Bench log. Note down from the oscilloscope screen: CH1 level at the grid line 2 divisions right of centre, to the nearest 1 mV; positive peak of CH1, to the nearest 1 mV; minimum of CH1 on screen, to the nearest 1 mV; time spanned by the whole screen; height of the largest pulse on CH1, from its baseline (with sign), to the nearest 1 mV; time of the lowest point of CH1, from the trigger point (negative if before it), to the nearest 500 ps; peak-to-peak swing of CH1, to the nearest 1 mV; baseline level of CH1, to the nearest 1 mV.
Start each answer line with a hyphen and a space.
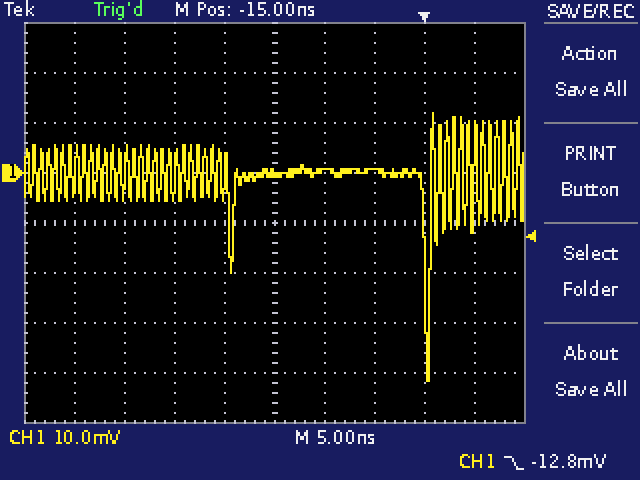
- 1 mV
- 12 mV
- -42 mV
- 50 ns
- -42 mV
- +500 ps
- 54 mV
- 0 mV
